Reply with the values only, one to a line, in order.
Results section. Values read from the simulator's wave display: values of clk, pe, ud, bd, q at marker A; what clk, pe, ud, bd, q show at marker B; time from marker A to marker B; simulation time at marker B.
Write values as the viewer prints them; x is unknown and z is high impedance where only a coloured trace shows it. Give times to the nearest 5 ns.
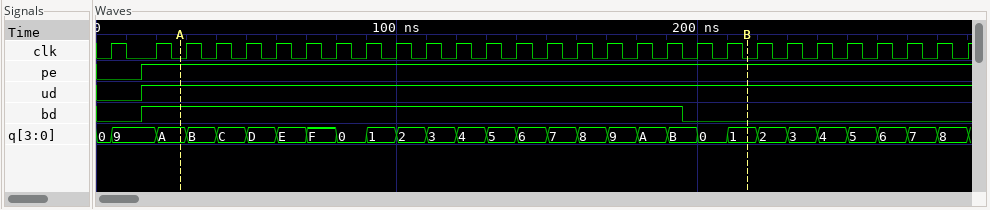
clk=0, pe=1, ud=1, bd=1, q=A
clk=0, pe=1, ud=1, bd=0, q=1
190 ns
215 ns
